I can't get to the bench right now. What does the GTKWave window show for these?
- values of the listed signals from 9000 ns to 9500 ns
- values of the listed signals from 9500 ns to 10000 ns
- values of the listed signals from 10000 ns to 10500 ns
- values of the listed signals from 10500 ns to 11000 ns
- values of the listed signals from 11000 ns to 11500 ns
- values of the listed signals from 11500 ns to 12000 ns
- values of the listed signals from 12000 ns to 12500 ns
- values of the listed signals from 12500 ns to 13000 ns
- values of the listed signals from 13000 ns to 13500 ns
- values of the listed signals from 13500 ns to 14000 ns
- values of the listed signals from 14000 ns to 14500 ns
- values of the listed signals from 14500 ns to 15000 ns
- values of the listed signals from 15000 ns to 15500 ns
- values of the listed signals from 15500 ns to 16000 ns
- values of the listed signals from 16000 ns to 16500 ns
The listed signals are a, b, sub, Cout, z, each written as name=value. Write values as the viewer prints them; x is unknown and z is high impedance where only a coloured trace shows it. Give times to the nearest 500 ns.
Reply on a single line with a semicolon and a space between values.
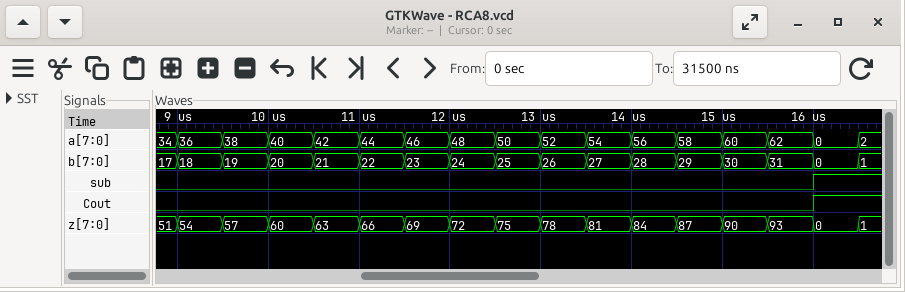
a=36, b=18, sub=0, Cout=0, z=54; a=38, b=19, sub=0, Cout=0, z=57; a=40, b=20, sub=0, Cout=0, z=60; a=42, b=21, sub=0, Cout=0, z=63; a=44, b=22, sub=0, Cout=0, z=66; a=46, b=23, sub=0, Cout=0, z=69; a=48, b=24, sub=0, Cout=0, z=72; a=50, b=25, sub=0, Cout=0, z=75; a=52, b=26, sub=0, Cout=0, z=78; a=54, b=27, sub=0, Cout=0, z=81; a=56, b=28, sub=0, Cout=0, z=84; a=58, b=29, sub=0, Cout=0, z=87; a=60, b=30, sub=0, Cout=0, z=90; a=62, b=31, sub=0, Cout=0, z=93; a=0, b=0, sub=1, Cout=1, z=0
